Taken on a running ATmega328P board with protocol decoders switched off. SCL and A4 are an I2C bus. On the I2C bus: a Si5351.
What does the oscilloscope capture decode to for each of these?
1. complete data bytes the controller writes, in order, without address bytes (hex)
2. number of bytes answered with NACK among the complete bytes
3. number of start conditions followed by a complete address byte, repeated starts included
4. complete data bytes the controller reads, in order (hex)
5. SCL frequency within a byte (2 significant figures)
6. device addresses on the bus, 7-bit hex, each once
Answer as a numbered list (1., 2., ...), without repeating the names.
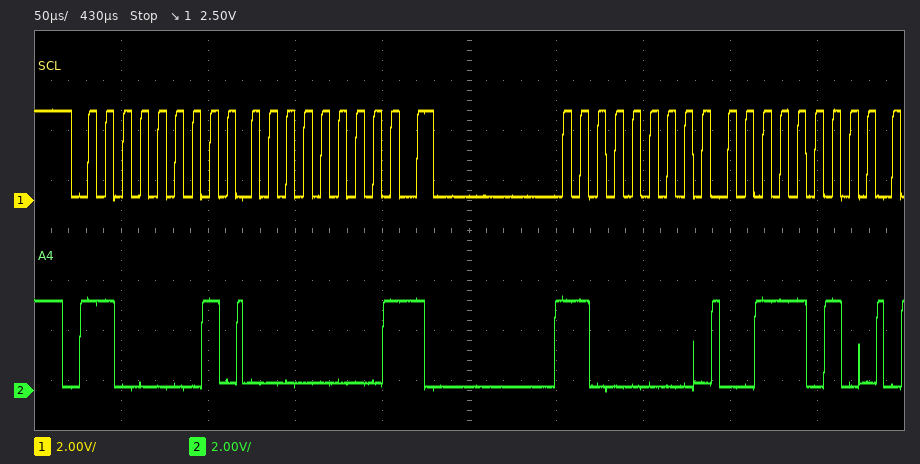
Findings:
1. 3A
2. 1
3. 2
4. 00
5. 100 kHz
6. 0x60
